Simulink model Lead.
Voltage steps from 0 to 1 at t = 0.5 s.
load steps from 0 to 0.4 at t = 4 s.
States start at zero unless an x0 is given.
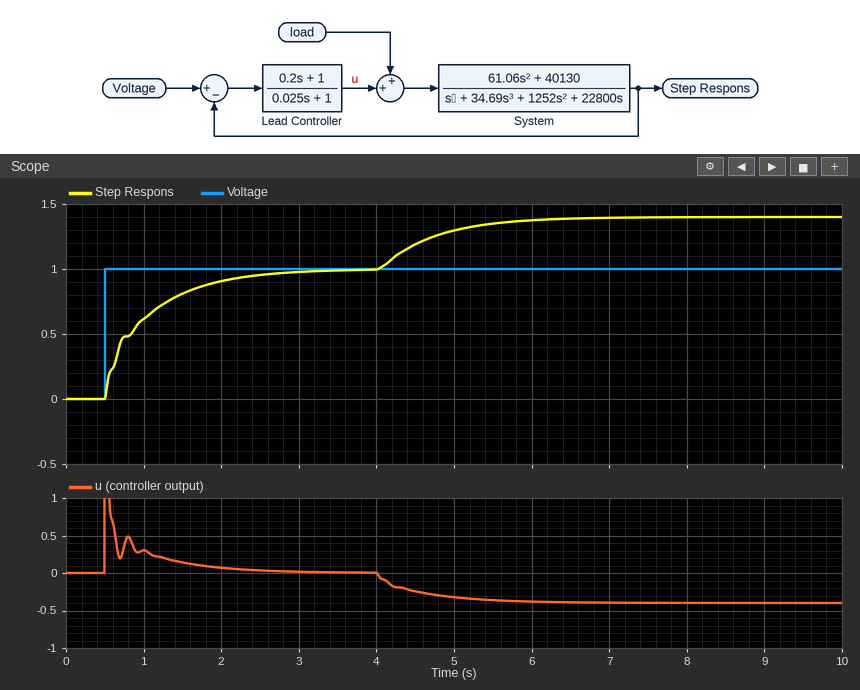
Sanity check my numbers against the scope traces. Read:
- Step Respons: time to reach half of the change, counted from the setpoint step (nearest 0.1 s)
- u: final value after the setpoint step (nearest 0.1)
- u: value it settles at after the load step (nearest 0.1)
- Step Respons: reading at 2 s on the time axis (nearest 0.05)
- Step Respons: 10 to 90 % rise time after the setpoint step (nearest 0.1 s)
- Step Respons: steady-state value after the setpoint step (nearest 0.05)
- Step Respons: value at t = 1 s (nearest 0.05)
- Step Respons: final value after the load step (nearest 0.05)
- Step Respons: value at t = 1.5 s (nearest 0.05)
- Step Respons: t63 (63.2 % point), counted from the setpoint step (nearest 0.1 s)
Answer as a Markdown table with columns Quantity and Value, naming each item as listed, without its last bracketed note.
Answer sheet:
| Quantity | Value |
|---|---|
| Step Respons: time to reach half of the change, counted from the setpoint step | 0.3 s |
| u: final value after the setpoint step | 0.0 |
| u: value it settles at after the load step | -0.4 |
| Step Respons: reading at 2 s on the time axis | 0.90 |
| Step Respons: 10 to 90 % rise time after the setpoint step | 1.4 s |
| Step Respons: steady-state value after the setpoint step | 1.00 |
| Step Respons: value at t = 1 s | 0.60 |
| Step Respons: final value after the load step | 1.40 |
| Step Respons: value at t = 1.5 s | 0.80 |
| Step Respons: t63 (63.2 % point), counted from the setpoint step | 0.5 s |
